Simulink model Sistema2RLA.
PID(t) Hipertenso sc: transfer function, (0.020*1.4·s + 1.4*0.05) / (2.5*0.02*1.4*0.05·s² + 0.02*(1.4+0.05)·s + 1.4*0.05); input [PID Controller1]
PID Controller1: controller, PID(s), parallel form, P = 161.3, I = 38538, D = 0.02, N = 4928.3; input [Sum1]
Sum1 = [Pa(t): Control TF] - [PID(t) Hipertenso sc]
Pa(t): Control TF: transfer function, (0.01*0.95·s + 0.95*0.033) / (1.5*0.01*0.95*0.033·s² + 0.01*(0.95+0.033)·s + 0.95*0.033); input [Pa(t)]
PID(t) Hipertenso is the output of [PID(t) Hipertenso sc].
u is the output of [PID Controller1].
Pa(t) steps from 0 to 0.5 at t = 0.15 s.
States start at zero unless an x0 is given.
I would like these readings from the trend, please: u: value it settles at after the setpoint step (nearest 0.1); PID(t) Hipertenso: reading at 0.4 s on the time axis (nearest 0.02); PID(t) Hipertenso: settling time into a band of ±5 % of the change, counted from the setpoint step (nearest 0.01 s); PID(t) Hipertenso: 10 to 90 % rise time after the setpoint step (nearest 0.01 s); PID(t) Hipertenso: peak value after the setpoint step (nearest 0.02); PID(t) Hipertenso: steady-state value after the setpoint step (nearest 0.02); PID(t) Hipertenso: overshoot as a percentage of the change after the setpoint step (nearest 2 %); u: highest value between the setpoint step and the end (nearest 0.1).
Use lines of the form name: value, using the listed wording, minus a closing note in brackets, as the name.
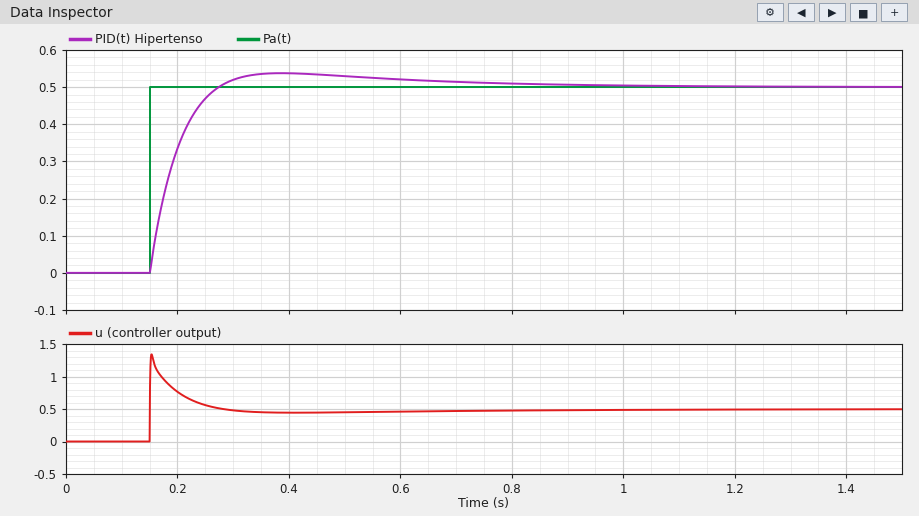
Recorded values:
u: value it settles at after the setpoint step: 0.5
PID(t) Hipertenso: reading at 0.4 s on the time axis: 0.54
PID(t) Hipertenso: settling time into a band of ±5 % of the change, counted from the setpoint step: 0.40 s
PID(t) Hipertenso: 10 to 90 % rise time after the setpoint step: 0.08 s
PID(t) Hipertenso: peak value after the setpoint step: 0.54
PID(t) Hipertenso: steady-state value after the setpoint step: 0.50
PID(t) Hipertenso: overshoot as a percentage of the change after the setpoint step: 8 %
u: highest value between the setpoint step and the end: 1.3
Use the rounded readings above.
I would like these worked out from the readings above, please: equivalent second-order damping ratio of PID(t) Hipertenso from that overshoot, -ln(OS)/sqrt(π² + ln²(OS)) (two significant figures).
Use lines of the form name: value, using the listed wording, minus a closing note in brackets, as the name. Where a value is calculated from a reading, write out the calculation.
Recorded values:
equivalent second-order damping ratio of PID(t) Hipertenso from that overshoot, -ln(OS)/sqrt(π² + ln²(OS)): ln(0.08) = -2.526; 2.526 / sqrt(9.870 + 6.379) = 0.63
